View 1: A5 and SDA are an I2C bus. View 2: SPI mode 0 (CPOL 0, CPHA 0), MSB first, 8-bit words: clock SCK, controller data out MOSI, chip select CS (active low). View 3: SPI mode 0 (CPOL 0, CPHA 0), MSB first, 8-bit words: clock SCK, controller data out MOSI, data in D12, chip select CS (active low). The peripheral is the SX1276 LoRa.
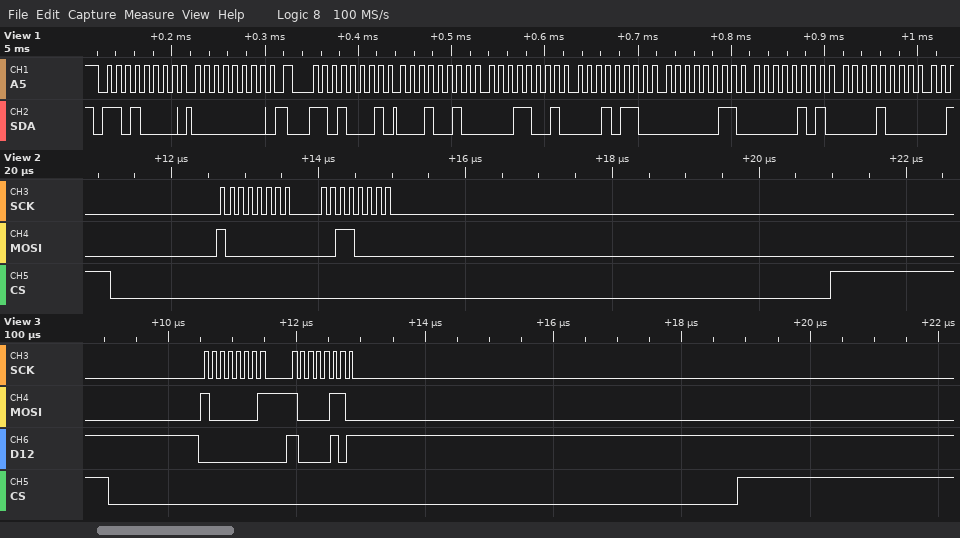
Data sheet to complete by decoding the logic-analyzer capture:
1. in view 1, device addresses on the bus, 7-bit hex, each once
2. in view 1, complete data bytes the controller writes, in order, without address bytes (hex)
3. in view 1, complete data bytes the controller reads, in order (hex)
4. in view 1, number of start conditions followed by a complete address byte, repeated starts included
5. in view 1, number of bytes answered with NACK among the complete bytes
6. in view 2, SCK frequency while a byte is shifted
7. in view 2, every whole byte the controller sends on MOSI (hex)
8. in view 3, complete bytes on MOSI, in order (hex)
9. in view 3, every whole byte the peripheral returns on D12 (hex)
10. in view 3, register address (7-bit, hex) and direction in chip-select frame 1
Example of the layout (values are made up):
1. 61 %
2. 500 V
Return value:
1. 0x68
2. 00
3. 12 19 16 03 05 08
4. 2
5. 0
6. 8 MHz
7. 0x80 0x30
8. 81 86
9. 00 85
10. 0x01 write
